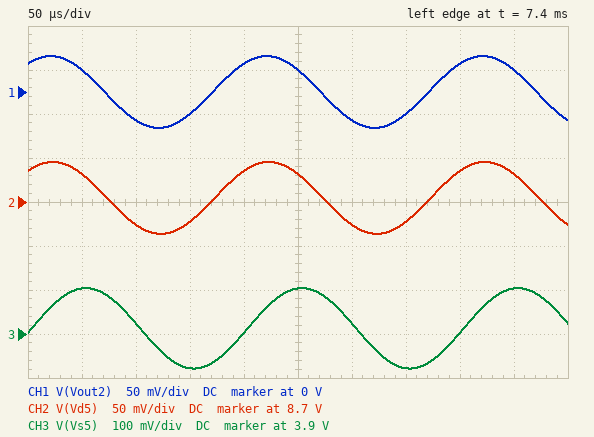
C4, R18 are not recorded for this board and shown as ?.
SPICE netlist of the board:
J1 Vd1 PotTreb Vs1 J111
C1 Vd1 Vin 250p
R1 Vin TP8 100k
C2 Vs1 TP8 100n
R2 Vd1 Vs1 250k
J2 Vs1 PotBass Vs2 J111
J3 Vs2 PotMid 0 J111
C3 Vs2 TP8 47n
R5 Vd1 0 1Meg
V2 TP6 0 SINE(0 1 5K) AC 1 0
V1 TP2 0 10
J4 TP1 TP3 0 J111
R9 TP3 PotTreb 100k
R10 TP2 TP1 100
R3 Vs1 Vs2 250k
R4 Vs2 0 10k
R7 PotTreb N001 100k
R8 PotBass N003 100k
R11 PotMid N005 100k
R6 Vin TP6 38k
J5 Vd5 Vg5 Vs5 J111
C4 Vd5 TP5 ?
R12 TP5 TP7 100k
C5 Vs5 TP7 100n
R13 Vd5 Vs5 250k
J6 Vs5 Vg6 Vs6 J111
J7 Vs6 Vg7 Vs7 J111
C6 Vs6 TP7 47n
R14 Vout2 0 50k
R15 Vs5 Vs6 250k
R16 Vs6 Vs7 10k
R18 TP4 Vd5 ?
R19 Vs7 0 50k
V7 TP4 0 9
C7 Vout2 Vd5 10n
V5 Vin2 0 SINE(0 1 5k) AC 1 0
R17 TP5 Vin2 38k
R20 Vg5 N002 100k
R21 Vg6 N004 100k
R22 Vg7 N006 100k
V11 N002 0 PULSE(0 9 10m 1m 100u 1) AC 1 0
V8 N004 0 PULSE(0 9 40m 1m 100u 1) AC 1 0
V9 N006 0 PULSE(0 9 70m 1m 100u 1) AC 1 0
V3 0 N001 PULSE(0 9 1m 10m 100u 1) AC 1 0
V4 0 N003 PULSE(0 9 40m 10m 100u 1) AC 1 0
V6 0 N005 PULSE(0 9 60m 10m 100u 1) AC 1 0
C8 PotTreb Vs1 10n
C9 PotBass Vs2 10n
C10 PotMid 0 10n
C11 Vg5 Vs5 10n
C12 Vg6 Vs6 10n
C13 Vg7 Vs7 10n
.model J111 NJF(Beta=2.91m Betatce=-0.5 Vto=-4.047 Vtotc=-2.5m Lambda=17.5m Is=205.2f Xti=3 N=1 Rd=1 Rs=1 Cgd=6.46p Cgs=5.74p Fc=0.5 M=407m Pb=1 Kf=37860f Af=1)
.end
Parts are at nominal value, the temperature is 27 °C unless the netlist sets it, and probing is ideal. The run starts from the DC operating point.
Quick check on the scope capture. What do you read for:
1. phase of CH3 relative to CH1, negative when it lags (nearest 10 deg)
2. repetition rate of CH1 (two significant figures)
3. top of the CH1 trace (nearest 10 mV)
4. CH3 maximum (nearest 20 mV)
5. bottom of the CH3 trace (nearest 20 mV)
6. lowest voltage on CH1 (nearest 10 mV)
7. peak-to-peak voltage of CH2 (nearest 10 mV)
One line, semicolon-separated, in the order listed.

-60 deg; 5.0 kHz; 40 mV; 4.00 V; 3.82 V; -40 mV; 80 mV
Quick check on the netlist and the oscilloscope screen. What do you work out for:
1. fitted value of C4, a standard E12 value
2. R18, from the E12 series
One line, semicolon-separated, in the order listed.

680 pF; 3.9 kΩ
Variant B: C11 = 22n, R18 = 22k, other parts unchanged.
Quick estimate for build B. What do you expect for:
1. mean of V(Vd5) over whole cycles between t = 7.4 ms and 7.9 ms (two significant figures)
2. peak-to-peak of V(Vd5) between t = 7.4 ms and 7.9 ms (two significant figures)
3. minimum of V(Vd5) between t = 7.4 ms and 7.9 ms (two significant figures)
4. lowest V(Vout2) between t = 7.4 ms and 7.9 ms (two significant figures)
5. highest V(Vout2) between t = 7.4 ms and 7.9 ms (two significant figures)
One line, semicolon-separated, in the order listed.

7.3 V; 320 mV; 7.2 V; -160 mV; 160 mV
